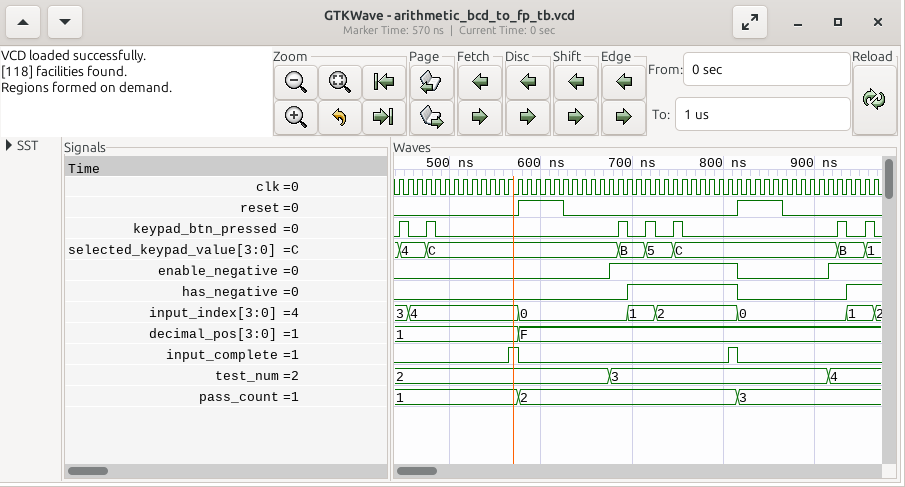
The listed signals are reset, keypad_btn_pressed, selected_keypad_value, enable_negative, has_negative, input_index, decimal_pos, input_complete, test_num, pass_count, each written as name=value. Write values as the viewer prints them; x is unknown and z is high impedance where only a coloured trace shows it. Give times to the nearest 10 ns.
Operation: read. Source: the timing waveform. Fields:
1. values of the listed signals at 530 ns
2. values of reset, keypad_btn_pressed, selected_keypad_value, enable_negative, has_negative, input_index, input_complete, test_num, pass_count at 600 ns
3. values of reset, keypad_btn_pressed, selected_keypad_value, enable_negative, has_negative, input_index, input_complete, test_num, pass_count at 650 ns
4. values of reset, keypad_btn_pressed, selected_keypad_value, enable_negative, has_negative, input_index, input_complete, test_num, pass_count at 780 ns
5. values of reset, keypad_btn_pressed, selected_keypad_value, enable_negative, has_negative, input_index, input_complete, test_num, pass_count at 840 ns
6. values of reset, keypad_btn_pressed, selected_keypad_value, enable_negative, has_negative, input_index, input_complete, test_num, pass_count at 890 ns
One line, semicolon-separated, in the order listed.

reset=0, keypad_btn_pressed=0, selected_keypad_value=C, enable_negative=0, has_negative=0, input_index=4, decimal_pos=1, input_complete=0, test_num=2, pass_count=1; reset=1, keypad_btn_pressed=0, selected_keypad_value=C, enable_negative=0, has_negative=0, input_index=0, input_complete=0, test_num=2, pass_count=2; reset=0, keypad_btn_pressed=0, selected_keypad_value=C, enable_negative=0, has_negative=0, input_index=0, input_complete=0, test_num=2, pass_count=2; reset=0, keypad_btn_pressed=0, selected_keypad_value=C, enable_negative=1, has_negative=1, input_index=2, input_complete=0, test_num=3, pass_count=2; reset=1, keypad_btn_pressed=0, selected_keypad_value=C, enable_negative=0, has_negative=0, input_index=0, input_complete=0, test_num=3, pass_count=3; reset=0, keypad_btn_pressed=0, selected_keypad_value=C, enable_negative=0, has_negative=0, input_index=0, input_complete=0, test_num=3, pass_count=3
